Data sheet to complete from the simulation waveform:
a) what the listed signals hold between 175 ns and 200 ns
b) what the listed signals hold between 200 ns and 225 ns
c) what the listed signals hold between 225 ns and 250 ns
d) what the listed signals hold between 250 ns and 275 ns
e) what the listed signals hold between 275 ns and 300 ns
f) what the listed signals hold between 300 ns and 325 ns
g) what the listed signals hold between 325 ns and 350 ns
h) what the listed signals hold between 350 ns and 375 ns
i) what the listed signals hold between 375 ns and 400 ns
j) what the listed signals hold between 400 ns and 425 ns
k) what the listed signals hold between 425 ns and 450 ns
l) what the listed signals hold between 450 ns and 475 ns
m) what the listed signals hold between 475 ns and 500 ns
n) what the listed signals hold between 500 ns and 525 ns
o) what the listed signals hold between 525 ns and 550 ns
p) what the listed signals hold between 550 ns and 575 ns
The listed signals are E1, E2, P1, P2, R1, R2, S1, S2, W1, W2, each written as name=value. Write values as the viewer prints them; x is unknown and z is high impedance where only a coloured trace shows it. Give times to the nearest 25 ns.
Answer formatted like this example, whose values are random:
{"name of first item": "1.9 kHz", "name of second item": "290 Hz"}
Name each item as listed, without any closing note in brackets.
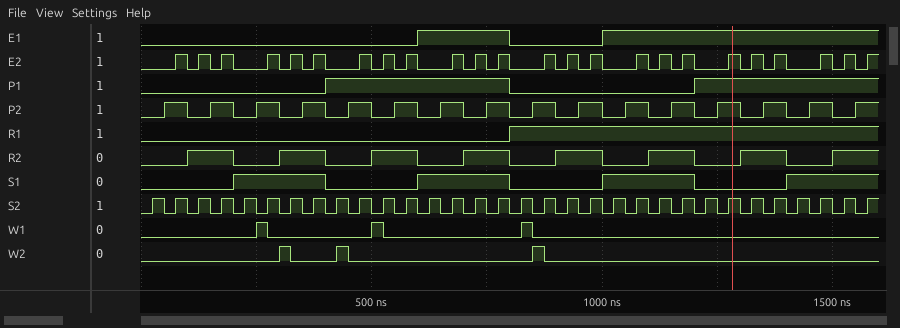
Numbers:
{"what the listed signals hold between 175 ns and 200 ns": "E1=0, E2=1, P1=0, P2=1, R1=0, R2=1, S1=0, S2=1, W1=0, W2=0", "what the listed signals hold between 200 ns and 225 ns": "E1=0, E2=0, P1=0, P2=0, R1=0, R2=0, S1=1, S2=0, W1=0, W2=0", "what the listed signals hold between 225 ns and 250 ns": "E1=0, E2=0, P1=0, P2=0, R1=0, R2=0, S1=1, S2=1, W1=0, W2=0", "what the listed signals hold between 250 ns and 275 ns": "E1=0, E2=0, P1=0, P2=1, R1=0, R2=0, S1=1, S2=0, W1=1, W2=0", "what the listed signals hold between 275 ns and 300 ns": "E1=0, E2=1, P1=0, P2=1, R1=0, R2=0, S1=1, S2=1, W1=0, W2=0", "what the listed signals hold between 300 ns and 325 ns": "E1=0, E2=0, P1=0, P2=0, R1=0, R2=1, S1=1, S2=0, W1=0, W2=1", "what the listed signals hold between 325 ns and 350 ns": "E1=0, E2=1, P1=0, P2=0, R1=0, R2=1, S1=1, S2=1, W1=0, W2=0", "what the listed signals hold between 350 ns and 375 ns": "E1=0, E2=0, P1=0, P2=1, R1=0, R2=1, S1=1, S2=0, W1=0, W2=0", "what the listed signals hold between 375 ns and 400 ns": "E1=0, E2=1, P1=0, P2=1, R1=0, R2=1, S1=1, S2=1, W1=0, W2=0", "what the listed signals hold between 400 ns and 425 ns": "E1=0, E2=0, P1=1, P2=0, R1=0, R2=0, S1=0, S2=0, W1=0, W2=0", "what the listed signals hold between 425 ns and 450 ns": "E1=0, E2=0, P1=1, P2=0, R1=0, R2=0, S1=0, S2=1, W1=0, W2=1", "what the listed signals hold between 450 ns and 475 ns": "E1=0, E2=0, P1=1, P2=1, R1=0, R2=0, S1=0, S2=0, W1=0, W2=0", "what the listed signals hold between 475 ns and 500 ns": "E1=0, E2=1, P1=1, P2=1, R1=0, R2=0, S1=0, S2=1, W1=0, W2=0", "what the listed signals hold between 500 ns and 525 ns": "E1=0, E2=0, P1=1, P2=0, R1=0, R2=1, S1=0, S2=0, W1=1, W2=0", "what the listed signals hold between 525 ns and 550 ns": "E1=0, E2=1, P1=1, P2=0, R1=0, R2=1, S1=0, S2=1, W1=0, W2=0", "what the listed signals hold between 550 ns and 575 ns": "E1=0, E2=0, P1=1, P2=1, R1=0, R2=1, S1=0, S2=0, W1=0, W2=0"}
